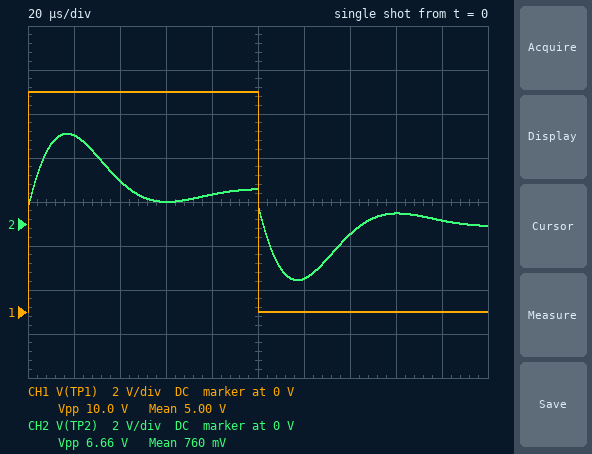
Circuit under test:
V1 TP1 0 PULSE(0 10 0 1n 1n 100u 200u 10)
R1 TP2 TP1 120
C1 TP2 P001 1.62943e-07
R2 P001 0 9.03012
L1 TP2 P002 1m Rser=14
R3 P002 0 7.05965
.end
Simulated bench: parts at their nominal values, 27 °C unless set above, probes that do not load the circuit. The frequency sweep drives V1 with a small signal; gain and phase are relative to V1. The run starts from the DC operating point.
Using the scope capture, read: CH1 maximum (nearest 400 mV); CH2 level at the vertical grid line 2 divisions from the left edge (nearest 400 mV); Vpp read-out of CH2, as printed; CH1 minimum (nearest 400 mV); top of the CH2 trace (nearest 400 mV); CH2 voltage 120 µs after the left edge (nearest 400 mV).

10.0 V
2.0 V
6.66 V
0 V
4.0 V
-2.4 V
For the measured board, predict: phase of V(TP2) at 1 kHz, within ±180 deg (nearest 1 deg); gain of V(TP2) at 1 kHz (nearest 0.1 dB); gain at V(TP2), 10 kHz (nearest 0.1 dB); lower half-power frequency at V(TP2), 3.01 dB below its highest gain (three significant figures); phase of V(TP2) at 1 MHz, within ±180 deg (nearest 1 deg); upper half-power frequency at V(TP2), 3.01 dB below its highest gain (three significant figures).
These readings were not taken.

13 deg
-16.1 dB
-4.9 dB
7.97 kHz
-6 deg
20.4 kHz
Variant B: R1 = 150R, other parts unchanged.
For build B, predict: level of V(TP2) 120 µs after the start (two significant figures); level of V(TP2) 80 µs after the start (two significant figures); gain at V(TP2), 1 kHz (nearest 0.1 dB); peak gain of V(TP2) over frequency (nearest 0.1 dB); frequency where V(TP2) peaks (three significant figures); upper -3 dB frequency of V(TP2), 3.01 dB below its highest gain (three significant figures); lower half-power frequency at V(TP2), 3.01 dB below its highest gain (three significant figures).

-2.2 V
1.1 V
-17.8 dB
-4.6 dB
12.8 kHz
19.3 kHz
8.35 kHz
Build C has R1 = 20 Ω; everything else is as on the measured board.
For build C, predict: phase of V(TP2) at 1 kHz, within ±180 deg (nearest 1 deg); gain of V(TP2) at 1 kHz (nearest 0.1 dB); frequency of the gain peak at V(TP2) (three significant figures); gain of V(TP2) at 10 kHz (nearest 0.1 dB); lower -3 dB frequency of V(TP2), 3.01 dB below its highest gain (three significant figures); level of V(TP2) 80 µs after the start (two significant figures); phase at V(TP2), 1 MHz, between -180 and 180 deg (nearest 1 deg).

7 deg
-5.5 dB
13.9 kHz
-1.0 dB
3.28 kHz
5.3 V
-4 deg
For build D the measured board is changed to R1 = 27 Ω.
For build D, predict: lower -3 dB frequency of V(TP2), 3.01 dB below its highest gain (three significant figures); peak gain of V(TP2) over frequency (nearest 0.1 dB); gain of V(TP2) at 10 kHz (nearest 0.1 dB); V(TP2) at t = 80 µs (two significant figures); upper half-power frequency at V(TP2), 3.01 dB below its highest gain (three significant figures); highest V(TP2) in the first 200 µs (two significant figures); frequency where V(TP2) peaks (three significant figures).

4.20 kHz
-1.0 dB
-1.3 dB
4.5 V
38.7 kHz
7.8 V
13.7 kHz
